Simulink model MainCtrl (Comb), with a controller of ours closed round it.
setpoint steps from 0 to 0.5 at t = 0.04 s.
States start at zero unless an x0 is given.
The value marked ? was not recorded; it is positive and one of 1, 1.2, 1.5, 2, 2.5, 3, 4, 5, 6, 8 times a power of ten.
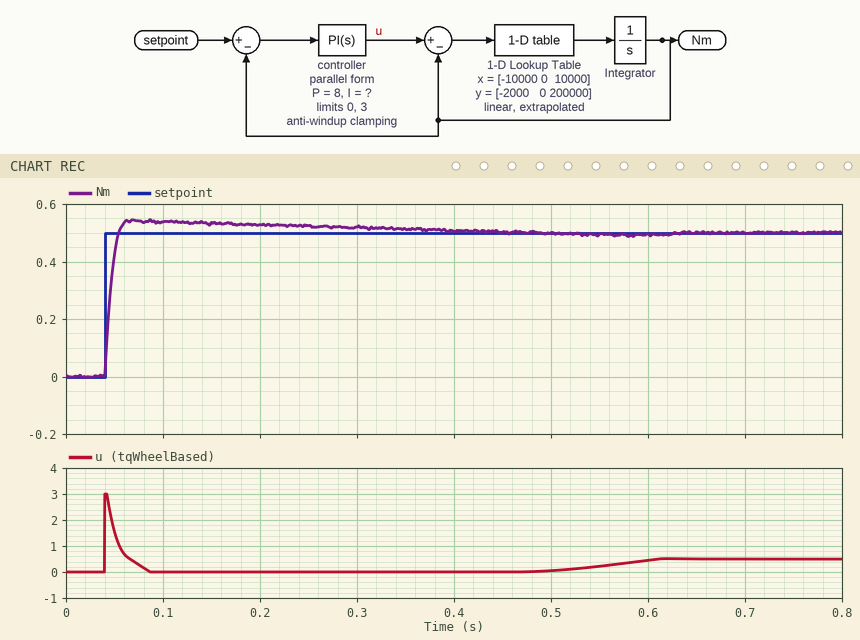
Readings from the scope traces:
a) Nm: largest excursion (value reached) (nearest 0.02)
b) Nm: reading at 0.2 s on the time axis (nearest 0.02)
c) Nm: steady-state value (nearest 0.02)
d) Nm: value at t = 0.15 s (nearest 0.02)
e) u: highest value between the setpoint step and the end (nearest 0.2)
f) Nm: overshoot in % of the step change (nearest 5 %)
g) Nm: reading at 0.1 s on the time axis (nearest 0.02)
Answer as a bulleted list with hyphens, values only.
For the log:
- 0.54
- 0.52
- 0.50
- 0.54
- 3.0
- 10 %
- 0.54
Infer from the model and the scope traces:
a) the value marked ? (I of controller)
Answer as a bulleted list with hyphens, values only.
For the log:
- 600
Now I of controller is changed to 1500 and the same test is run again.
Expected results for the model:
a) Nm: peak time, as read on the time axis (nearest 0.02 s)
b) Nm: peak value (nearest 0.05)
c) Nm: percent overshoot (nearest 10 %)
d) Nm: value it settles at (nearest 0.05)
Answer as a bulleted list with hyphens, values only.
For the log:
- 0.06 s
- 0.60
- 20 %
- 0.50
